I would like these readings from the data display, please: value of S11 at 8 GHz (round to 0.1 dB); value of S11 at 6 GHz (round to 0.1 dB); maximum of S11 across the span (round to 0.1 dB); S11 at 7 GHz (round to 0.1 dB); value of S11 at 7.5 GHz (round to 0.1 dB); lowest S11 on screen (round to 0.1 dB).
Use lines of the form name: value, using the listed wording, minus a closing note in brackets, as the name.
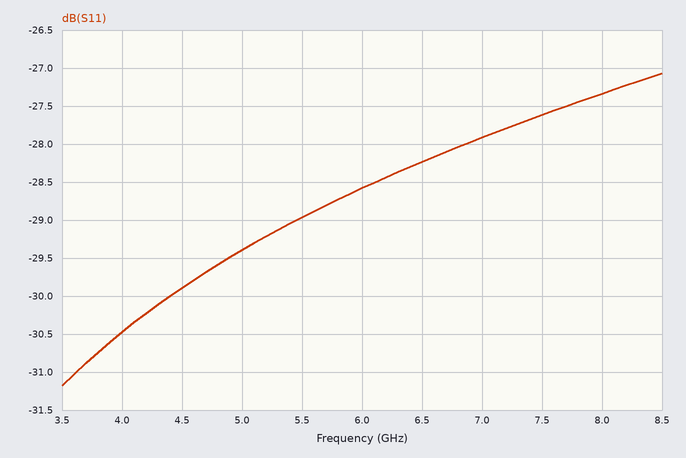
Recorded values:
value of S11 at 8 GHz: -27.3 dB
value of S11 at 6 GHz: -28.6 dB
maximum of S11 across the span: -27.1 dB
S11 at 7 GHz: -27.9 dB
value of S11 at 7.5 GHz: -27.6 dB
lowest S11 on screen: -31.2 dB
